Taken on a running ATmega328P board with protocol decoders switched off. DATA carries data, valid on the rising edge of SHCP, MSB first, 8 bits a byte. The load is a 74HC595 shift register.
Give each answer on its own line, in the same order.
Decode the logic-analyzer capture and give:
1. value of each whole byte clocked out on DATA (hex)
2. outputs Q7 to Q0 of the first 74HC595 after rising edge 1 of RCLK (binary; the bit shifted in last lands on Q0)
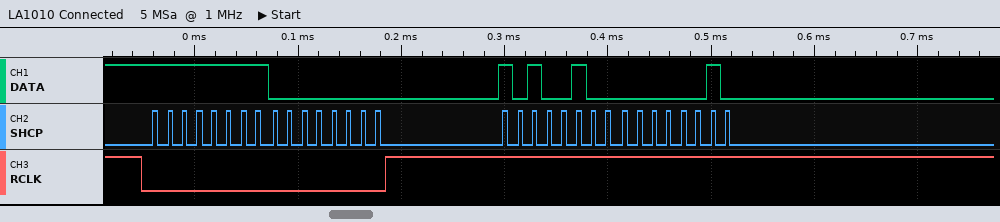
FF 00 A4 02
00000000
